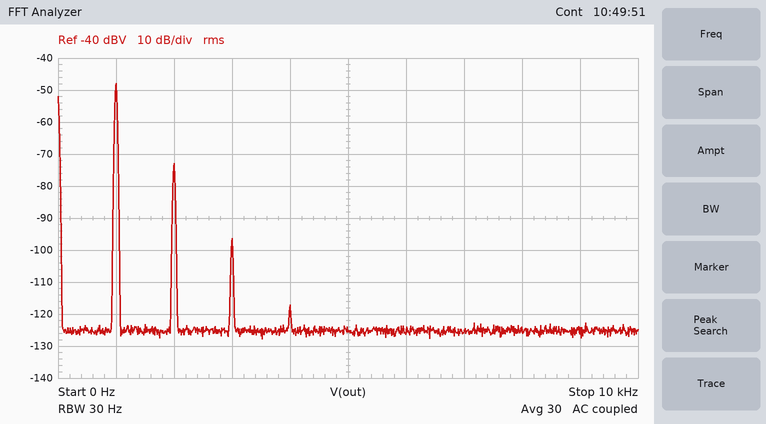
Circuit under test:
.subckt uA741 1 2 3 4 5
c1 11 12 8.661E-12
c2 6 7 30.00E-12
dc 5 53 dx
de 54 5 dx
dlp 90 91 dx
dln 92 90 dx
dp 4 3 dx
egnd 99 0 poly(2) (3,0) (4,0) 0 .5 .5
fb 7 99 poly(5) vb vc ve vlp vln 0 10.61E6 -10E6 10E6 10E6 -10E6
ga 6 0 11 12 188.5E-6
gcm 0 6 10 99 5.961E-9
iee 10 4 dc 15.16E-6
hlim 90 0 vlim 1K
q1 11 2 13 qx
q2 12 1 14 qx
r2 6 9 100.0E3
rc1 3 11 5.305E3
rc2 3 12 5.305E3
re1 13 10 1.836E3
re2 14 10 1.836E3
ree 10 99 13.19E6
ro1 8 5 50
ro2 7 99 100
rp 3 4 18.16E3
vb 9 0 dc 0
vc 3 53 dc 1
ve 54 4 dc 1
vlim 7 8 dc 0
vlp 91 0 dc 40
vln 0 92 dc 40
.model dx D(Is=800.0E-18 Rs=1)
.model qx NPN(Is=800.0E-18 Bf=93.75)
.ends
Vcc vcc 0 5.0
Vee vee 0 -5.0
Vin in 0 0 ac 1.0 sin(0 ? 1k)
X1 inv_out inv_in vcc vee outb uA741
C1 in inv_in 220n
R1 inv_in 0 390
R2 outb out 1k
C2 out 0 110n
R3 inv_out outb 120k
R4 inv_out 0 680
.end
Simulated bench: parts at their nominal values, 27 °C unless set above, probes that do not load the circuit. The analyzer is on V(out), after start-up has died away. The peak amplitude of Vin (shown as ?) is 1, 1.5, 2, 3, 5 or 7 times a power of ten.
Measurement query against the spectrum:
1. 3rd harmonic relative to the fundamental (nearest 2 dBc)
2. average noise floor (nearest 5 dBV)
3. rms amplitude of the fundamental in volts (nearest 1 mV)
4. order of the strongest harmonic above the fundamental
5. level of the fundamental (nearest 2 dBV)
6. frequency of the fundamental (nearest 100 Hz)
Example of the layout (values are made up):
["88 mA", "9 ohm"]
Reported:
["-48 dBc", "-125 dBV", "4 mV", "2", "-48 dBV", "1.0 kHz"]
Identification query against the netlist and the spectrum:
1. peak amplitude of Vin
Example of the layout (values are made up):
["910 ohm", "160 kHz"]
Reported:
["15 mV"]
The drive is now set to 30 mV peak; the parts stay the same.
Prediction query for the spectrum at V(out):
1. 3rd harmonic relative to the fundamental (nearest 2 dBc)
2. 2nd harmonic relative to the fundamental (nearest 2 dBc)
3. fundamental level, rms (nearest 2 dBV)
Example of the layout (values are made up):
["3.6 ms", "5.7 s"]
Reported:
["-36 dBc", "-18 dBc", "-42 dBV"]
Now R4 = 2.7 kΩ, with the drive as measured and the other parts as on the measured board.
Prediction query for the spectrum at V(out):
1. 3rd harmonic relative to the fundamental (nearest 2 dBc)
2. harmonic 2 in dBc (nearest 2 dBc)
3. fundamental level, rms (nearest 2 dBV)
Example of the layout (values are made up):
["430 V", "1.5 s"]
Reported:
["-60 dBc", "-28 dBc", "-68 dBV"]
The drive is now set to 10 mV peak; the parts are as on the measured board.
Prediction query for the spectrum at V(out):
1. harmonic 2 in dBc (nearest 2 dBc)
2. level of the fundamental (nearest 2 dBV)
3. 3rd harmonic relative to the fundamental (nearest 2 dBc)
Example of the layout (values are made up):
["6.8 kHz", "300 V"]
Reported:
["-28 dBc", "-52 dBV", "-56 dBc"]
